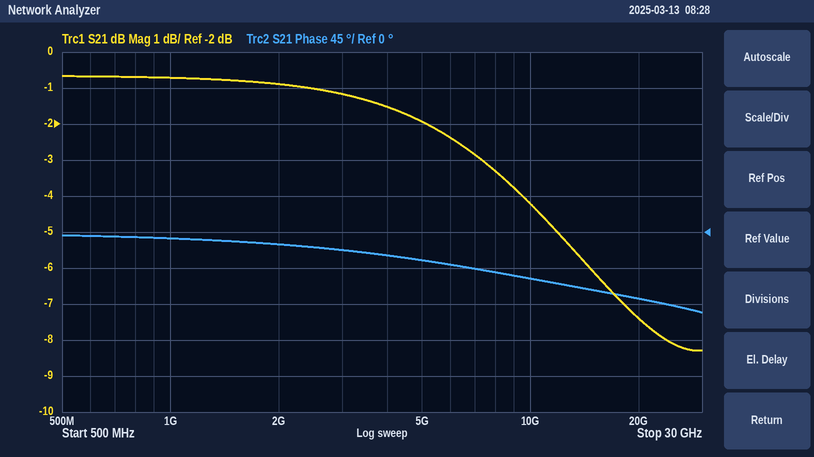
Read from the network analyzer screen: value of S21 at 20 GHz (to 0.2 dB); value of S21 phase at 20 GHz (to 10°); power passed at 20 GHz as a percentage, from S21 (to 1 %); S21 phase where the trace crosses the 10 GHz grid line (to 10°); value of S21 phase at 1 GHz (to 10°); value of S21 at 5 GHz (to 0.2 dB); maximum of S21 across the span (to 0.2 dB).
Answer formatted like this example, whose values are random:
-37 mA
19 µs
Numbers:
-7.4 dB
-80°
18 %
-60°
-10°
-2.0 dB
-0.6 dB
